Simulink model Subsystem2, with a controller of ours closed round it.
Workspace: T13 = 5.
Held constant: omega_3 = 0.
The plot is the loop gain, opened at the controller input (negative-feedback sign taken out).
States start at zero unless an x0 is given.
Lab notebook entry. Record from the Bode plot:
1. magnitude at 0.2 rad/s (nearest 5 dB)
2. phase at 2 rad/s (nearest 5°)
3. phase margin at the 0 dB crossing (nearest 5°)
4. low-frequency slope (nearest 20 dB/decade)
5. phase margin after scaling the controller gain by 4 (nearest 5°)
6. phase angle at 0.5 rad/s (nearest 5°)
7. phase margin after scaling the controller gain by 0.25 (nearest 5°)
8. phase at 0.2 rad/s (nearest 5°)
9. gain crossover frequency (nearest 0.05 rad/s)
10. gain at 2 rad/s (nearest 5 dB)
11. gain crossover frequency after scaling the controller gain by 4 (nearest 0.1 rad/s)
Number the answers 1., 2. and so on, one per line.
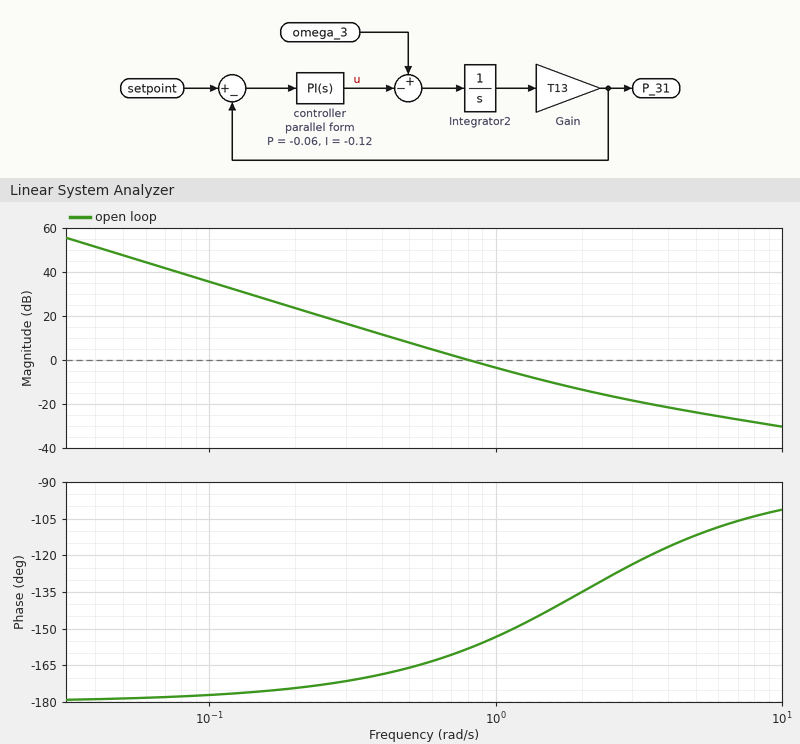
1. 25 dB
2. -135°
3. 20°
4. -40 dB/decade
5. 40°
6. -165°
7. 10°
8. -175°
9. 0.80 rad/s
10. -15 dB
11. 1.8 rad/s
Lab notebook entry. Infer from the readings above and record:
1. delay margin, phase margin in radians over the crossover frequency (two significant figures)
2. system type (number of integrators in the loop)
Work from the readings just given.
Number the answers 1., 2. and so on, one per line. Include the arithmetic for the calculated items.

1. 20 × π / 180 / 0.8 = 0.44 s
2. 2
